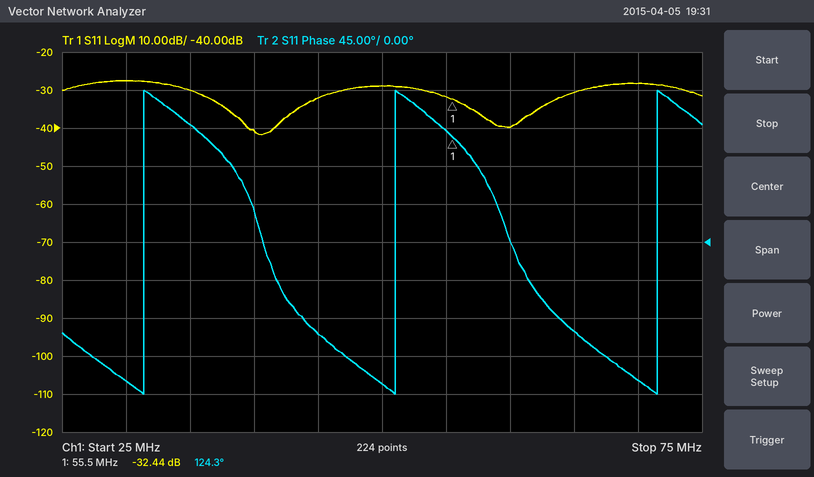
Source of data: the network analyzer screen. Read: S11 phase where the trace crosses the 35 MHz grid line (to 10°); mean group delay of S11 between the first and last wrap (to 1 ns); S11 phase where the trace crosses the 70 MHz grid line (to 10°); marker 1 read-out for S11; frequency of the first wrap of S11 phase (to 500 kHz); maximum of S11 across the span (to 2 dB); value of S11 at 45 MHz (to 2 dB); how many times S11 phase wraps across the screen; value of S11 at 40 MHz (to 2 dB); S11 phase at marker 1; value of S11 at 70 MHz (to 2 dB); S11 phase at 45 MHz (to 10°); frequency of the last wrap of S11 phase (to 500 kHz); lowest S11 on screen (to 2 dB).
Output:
140°
50 ns
-160°
-32.44 dB
31.5 MHz
-28 dB
-32 dB
3
-40 dB
124.3°
-28 dB
-110°
71.5 MHz
-42 dB
